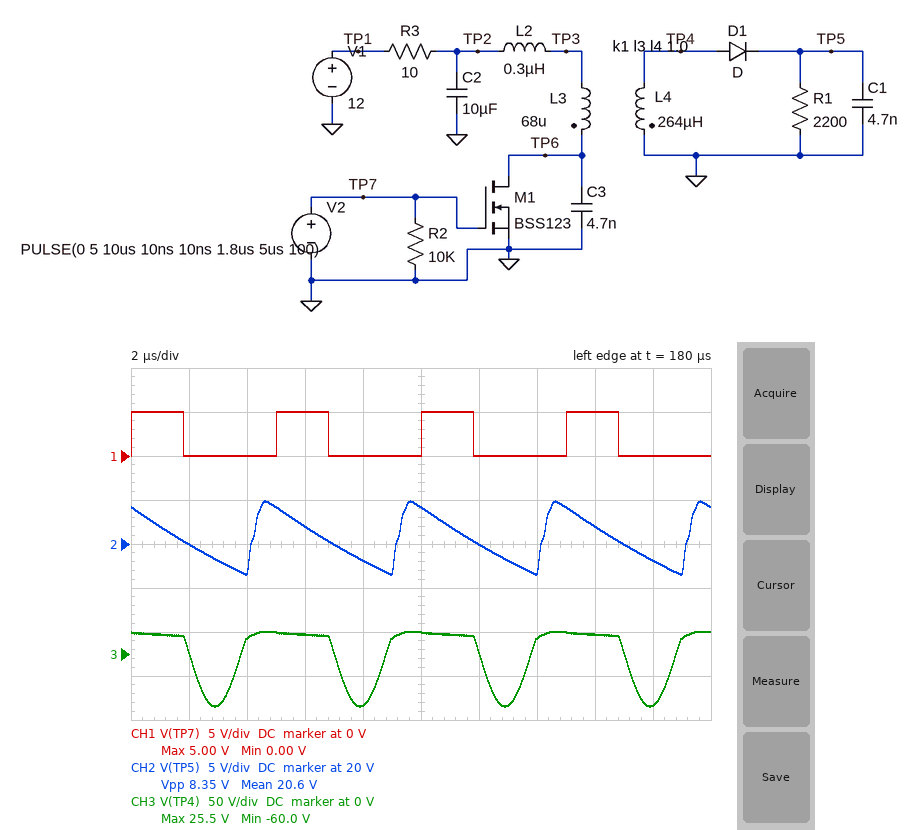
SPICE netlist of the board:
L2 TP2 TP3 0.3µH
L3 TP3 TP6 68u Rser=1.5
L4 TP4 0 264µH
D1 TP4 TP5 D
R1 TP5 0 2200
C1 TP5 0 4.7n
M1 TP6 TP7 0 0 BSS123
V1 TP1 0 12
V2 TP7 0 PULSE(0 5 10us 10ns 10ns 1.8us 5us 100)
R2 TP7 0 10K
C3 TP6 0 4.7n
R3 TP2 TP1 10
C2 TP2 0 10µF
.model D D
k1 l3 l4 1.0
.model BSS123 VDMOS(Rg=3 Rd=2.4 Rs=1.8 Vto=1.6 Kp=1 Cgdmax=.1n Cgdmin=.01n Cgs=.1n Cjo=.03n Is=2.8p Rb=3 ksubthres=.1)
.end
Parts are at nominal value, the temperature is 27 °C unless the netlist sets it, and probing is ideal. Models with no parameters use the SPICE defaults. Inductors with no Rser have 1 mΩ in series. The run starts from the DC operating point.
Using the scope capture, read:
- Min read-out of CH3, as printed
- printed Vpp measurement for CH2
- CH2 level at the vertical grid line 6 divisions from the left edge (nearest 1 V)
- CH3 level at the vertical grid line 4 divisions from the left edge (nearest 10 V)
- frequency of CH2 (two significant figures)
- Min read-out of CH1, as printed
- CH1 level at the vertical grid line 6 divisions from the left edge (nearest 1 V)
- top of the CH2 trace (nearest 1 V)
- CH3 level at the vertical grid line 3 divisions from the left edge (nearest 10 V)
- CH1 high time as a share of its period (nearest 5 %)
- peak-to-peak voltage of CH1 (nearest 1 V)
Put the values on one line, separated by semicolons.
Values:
-60.0 V; 8.35 V; 20 V; -60 V; 200 kHz; 0.00 V; 0 V; 25 V; 20 V; 35 %; 5 V
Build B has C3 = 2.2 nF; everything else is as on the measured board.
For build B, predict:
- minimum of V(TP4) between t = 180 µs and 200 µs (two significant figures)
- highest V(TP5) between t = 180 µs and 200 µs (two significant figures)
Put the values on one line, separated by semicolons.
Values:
-110 V; 26 V
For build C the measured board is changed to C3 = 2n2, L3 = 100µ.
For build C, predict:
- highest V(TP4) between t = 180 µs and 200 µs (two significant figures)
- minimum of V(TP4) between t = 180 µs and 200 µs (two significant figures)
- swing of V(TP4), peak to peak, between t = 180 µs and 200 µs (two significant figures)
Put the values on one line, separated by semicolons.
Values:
21 V; -69 V; 90 V
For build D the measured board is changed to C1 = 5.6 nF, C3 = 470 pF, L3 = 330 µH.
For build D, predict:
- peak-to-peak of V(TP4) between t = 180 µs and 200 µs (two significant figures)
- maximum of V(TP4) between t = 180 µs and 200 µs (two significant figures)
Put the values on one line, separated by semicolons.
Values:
61 V; 12 V
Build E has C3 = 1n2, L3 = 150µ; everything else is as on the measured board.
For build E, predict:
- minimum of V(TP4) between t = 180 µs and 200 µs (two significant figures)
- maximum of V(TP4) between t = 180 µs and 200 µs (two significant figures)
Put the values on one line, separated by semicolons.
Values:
-66 V; 17 V
